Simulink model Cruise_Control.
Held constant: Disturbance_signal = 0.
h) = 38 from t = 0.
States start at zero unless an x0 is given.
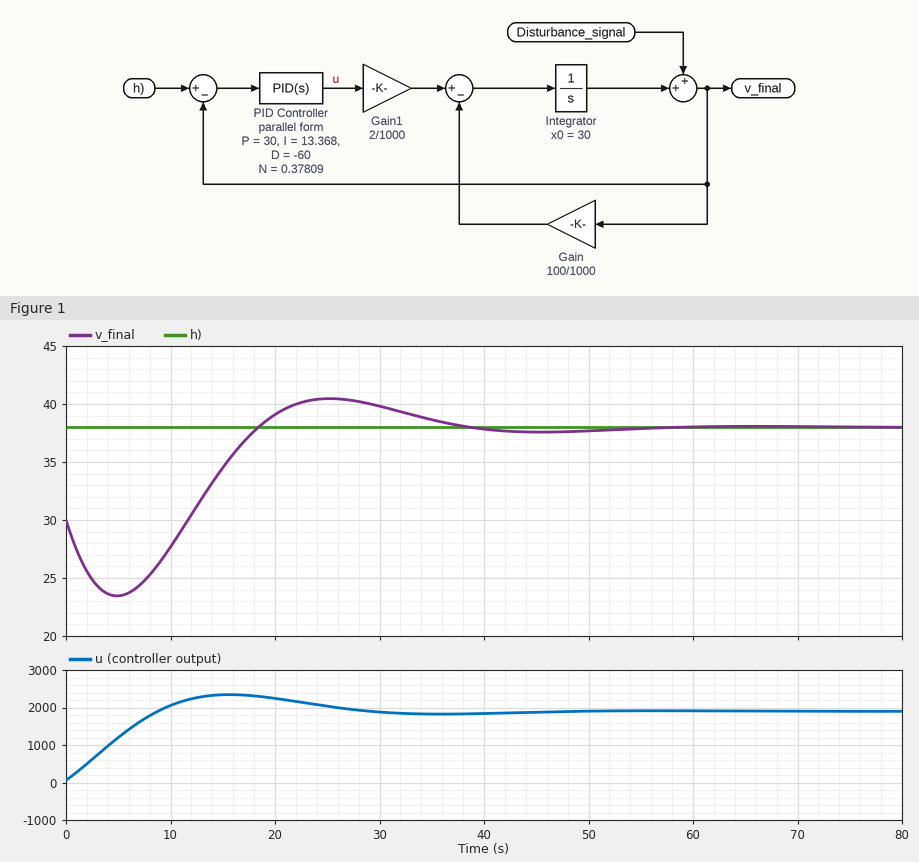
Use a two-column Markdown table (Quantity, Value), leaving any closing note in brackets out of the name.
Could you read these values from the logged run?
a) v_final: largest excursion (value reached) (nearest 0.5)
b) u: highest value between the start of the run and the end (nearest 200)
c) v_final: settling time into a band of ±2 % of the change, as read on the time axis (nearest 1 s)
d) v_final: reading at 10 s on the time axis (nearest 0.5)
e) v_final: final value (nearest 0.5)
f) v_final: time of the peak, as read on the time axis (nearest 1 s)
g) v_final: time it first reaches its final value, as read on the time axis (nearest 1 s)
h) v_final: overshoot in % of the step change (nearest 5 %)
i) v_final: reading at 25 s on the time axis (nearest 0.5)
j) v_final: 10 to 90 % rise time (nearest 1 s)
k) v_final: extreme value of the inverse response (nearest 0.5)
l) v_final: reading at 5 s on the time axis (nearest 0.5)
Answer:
| Quantity | Value |
|---|---|
| v_final: largest excursion (value reached) | 40.5 |
| u: highest value between the start of the run and the end | 2400 |
| v_final: settling time into a band of ±2 % of the change, as read on the time axis | 54 s |
| v_final: reading at 10 s on the time axis | 27.5 |
| v_final: final value | 38.0 |
| v_final: time of the peak, as read on the time axis | 25 s |
| v_final: time it first reaches its final value, as read on the time axis | 18 s |
| v_final: overshoot in % of the step change | 30 % |
| v_final: reading at 25 s on the time axis | 40.5 |
| v_final: 10 to 90 % rise time | 5 s |
| v_final: extreme value of the inverse response | 23.5 |
| v_final: reading at 5 s on the time axis | 23.5 |
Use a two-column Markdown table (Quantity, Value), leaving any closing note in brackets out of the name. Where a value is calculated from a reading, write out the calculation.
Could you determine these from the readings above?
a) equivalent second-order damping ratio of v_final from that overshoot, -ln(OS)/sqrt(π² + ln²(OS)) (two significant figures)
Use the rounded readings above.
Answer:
| Quantity | Value |
|---|---|
| equivalent second-order damping ratio of v_final from that overshoot, -ln(OS)/sqrt(π² + ln²(OS)) | ln(0.3) = -1.204; 1.204 / sqrt(9.870 + 1.450) = 0.36 |
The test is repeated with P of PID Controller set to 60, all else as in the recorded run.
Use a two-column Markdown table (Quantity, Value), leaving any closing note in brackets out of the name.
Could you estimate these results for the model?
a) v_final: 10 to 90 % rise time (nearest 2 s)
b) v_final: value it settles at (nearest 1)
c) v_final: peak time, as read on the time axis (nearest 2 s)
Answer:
| Quantity | Value |
|---|---|
| v_final: 10 to 90 % rise time | 8 s |
| v_final: value it settles at | 38 |
| v_final: peak time, as read on the time axis | 28 s |
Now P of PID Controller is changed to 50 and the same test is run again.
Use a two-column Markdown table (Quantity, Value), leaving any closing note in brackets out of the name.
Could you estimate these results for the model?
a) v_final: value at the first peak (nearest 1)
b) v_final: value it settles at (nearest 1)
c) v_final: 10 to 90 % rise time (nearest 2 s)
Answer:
| Quantity | Value |
|---|---|
| v_final: value at the first peak | 39 |
| v_final: value it settles at | 38 |
| v_final: 10 to 90 % rise time | 8 s |
